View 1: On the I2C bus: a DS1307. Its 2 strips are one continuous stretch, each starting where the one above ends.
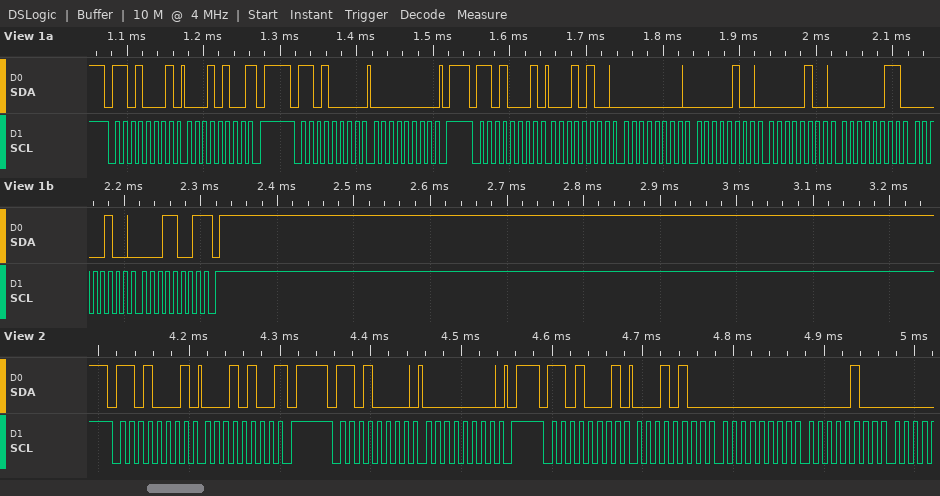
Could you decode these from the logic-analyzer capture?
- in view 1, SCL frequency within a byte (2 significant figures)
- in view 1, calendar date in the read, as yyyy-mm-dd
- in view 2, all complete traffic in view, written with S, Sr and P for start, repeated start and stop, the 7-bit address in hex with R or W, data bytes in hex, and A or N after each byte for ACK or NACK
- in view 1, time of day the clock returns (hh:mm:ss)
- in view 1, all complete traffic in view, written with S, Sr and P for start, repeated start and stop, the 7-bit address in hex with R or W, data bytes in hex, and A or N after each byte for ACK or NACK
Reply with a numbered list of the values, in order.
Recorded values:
1. 100 kHz
2. 2019-04-03
3. S 68R A 14 N P S 68W A 00 A P S 68R A 14 A 00 A 04 A
4. 04:00:14
5. S 68R A 14 N P S 68W A 00 A P S 68R A 14 A 00 A 04 A 04 A 03 A 04 A 19 N P
